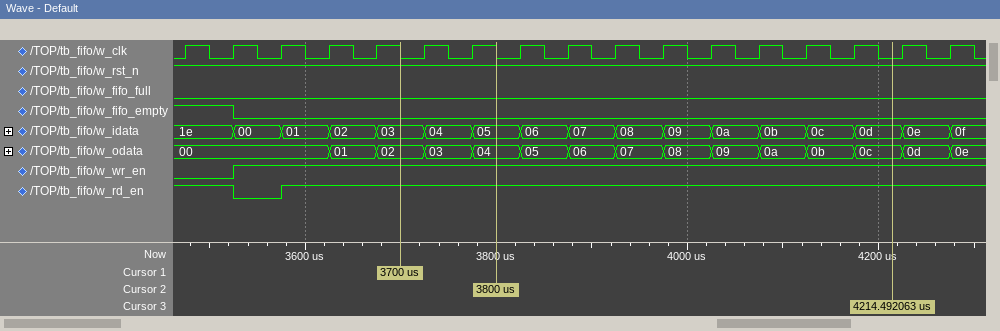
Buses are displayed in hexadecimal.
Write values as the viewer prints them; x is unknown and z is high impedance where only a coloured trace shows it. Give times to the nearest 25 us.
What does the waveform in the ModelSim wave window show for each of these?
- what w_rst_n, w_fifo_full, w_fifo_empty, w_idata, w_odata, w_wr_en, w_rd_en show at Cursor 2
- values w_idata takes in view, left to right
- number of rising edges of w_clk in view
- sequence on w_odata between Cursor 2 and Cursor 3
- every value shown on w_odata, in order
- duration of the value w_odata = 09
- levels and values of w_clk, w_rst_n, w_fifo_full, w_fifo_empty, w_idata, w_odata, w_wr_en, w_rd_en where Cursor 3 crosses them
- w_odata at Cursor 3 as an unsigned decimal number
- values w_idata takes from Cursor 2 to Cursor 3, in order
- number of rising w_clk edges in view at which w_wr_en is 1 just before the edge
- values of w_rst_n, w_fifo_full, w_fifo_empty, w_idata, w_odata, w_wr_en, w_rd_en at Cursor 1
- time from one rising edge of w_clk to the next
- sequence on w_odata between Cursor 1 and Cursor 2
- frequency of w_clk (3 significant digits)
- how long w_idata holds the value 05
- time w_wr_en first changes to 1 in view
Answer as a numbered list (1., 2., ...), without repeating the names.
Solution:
1. w_rst_n=1, w_fifo_full=0, w_fifo_empty=0, w_idata=05, w_odata=04, w_wr_en=1, w_rd_en=1
2. 1e, 00, 01, 02, 03, 04, 05, 06, 07, 08, 09, 0a, 0b, 0c, 0d, 0e, 0f
3. 17
4. 04, 05, 06, 07, 08, 09, 0a, 0b, 0c
5. 00, 01, 02, 03, 04, 05, 06, 07, 08, 09, 0a, 0b, 0c, 0d, 0e
6. 50 us
7. w_clk=0, w_rst_n=1, w_fifo_full=0, w_fifo_empty=0, w_idata=0d, w_odata=0c, w_wr_en=1, w_rd_en=1
8. 12
9. 05, 06, 07, 08, 09, 0a, 0b, 0c, 0d
10. 15
11. w_rst_n=1, w_fifo_full=0, w_fifo_empty=0, w_idata=03, w_odata=02, w_wr_en=1, w_rd_en=1
12. 50 us
13. 02, 03, 04
14. 20.0 kHz
15. 50 us
16. 3525 us
